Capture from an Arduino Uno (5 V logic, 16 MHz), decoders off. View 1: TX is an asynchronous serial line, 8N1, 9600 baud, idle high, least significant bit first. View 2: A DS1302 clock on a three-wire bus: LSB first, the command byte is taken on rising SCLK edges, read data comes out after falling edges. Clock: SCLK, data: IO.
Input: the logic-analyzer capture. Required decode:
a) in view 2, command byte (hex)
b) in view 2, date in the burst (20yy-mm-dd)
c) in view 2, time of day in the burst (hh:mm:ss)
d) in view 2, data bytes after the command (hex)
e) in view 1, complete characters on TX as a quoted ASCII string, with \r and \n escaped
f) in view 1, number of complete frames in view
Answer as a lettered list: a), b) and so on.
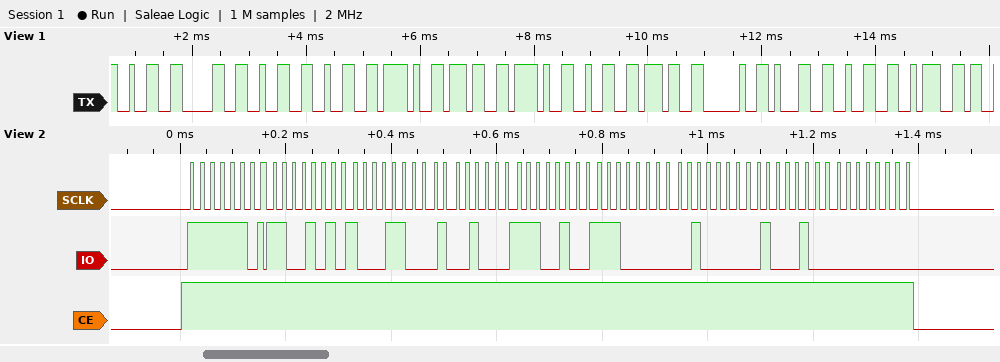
a) 0xBF
b) 2022-07-27
c) 12:31:53
d) 53 31 12 27 07 04 22 00
e) "2022/7/27 12:"
f) 13
